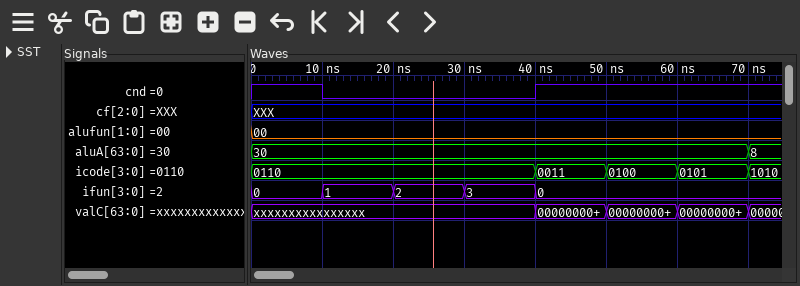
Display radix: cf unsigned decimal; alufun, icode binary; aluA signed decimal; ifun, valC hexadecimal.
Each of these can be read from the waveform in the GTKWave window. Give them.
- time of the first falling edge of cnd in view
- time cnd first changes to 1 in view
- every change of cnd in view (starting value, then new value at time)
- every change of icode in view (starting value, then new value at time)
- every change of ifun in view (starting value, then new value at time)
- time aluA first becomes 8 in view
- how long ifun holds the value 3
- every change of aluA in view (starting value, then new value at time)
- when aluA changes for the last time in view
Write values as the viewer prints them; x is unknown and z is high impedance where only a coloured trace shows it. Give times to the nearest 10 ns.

10 ns
40 ns
1, 0 at 10 ns, 1 at 40 ns
0110, 0011 at 40 ns, 0100 at 50 ns, 0101 at 60 ns, 1010 at 70 ns
0, 1 at 10 ns, 2 at 20 ns, 3 at 30 ns, 0 at 40 ns
70 ns
10 ns
30, 8 at 70 ns
70 ns
